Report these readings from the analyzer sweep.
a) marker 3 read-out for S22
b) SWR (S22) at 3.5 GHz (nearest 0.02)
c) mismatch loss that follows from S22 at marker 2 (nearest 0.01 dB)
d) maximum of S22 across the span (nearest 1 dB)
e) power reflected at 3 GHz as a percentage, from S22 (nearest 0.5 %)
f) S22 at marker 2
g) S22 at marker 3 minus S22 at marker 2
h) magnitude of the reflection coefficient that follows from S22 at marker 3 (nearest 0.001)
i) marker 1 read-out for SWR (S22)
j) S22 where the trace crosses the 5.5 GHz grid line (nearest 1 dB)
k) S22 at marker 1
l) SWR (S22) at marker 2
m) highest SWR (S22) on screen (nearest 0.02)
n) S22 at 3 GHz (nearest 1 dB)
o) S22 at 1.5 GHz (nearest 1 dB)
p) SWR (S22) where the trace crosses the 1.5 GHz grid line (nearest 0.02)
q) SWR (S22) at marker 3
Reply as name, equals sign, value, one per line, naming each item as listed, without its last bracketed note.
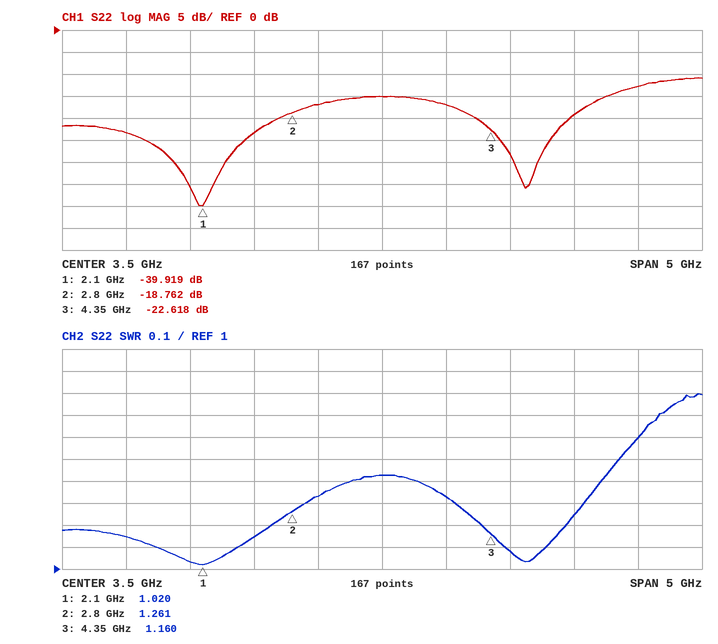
marker 3 read-out for S22 = -22.618 dB
SWR (S22) at 3.5 GHz = 1.42
mismatch loss that follows from S22 at marker 2 = 0.06 dB
maximum of S22 across the span = -11 dB
power reflected at 3 GHz as a percentage, from S22 = 2.0 %
S22 at marker 2 = -18.762 dB
S22 at marker 3 minus S22 at marker 2 = -3.856 dB
magnitude of the reflection coefficient that follows from S22 at marker 3 = 0.074
marker 1 read-out for SWR = 1.020
S22 where the trace crosses the 5.5 GHz grid line = -13 dB
S22 at marker 1 = -39.919 dB
SWR (S22) at marker 2 = 1.261
highest SWR (S22) on screen = 1.80
S22 at 3 GHz = -17 dB
S22 at 1.5 GHz = -23 dB
SWR (S22) where the trace crosses the 1.5 GHz grid line = 1.14
SWR (S22) at marker 3 = 1.160
